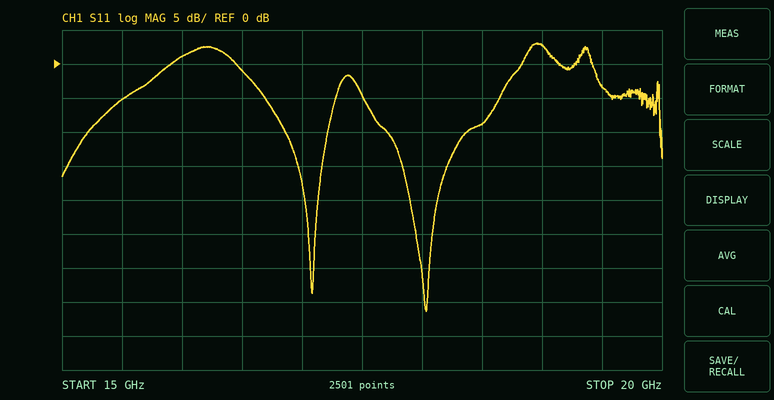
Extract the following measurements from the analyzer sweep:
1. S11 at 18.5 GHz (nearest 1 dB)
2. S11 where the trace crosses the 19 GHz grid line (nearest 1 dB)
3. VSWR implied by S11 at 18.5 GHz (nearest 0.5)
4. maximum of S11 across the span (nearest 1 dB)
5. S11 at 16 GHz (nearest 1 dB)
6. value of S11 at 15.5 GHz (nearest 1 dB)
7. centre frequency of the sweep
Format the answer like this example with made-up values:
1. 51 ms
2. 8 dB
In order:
1. -9 dB
2. 3 dB
3. 2.0
4. 3 dB
5. 1 dB
6. -5 dB
7. 17.5 GHz
